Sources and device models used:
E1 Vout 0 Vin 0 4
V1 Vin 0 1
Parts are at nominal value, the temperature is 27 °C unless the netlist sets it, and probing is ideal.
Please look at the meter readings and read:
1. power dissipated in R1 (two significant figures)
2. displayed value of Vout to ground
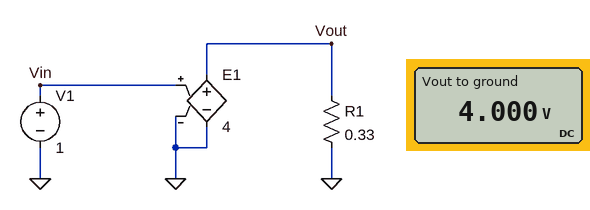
48 W
4.000 V
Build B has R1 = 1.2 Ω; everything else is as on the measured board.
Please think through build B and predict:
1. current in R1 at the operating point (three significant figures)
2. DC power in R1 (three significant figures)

3.33 A
13.3 W
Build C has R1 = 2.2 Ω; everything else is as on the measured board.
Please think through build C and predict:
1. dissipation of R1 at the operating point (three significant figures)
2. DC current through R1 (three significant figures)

7.27 W
1.82 A
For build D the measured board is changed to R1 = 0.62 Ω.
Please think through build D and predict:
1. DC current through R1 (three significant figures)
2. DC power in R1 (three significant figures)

6.45 A
25.8 W
